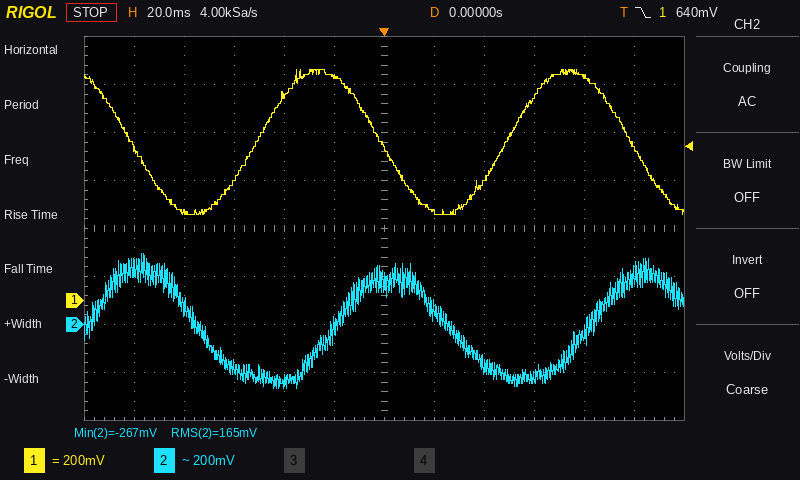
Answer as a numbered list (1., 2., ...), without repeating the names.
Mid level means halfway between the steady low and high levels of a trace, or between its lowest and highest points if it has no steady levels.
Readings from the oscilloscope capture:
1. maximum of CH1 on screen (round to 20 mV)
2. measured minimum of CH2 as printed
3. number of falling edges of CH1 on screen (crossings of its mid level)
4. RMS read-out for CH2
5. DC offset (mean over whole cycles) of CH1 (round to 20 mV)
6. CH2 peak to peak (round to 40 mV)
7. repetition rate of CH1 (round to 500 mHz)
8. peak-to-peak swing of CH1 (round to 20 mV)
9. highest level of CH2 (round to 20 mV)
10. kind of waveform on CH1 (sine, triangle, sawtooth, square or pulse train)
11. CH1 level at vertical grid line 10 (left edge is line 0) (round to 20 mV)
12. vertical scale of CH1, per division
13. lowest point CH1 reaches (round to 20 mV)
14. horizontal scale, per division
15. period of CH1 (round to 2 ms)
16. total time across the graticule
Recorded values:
1. 960 mV
2. -267 mV
3. 3
4. 165 mV
5. 660 mV
6. 560 mV
7. 10.0 Hz
8. 600 mV
9. 300 mV
10. sine
11. 940 mV
12. 200 mV
13. 360 mV
14. 20 ms
15. 100 ms
16. 240 ms
